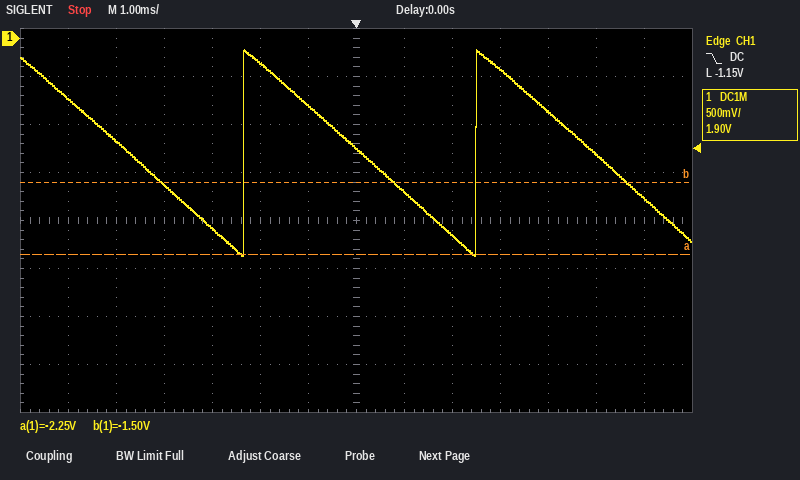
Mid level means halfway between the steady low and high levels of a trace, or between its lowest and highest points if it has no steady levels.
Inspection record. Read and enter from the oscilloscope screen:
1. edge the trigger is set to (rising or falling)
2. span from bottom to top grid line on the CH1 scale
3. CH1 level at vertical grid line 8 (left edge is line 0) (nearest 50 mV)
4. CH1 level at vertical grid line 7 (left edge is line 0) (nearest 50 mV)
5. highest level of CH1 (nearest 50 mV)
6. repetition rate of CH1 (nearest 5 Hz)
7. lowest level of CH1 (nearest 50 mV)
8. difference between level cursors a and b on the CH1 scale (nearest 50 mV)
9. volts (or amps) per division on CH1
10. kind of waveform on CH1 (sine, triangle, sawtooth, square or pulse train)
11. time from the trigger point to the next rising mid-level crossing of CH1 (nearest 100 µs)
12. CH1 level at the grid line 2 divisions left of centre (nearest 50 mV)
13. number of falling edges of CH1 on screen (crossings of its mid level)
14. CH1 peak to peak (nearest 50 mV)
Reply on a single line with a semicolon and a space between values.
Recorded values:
falling; 4 V; -1.60 V; -1.15 V; -100 mV; 205 Hz; -2.25 V; 750 mV; 500 mV; sawtooth; 2.5 ms; -250 mV; 3; 2.15 V
